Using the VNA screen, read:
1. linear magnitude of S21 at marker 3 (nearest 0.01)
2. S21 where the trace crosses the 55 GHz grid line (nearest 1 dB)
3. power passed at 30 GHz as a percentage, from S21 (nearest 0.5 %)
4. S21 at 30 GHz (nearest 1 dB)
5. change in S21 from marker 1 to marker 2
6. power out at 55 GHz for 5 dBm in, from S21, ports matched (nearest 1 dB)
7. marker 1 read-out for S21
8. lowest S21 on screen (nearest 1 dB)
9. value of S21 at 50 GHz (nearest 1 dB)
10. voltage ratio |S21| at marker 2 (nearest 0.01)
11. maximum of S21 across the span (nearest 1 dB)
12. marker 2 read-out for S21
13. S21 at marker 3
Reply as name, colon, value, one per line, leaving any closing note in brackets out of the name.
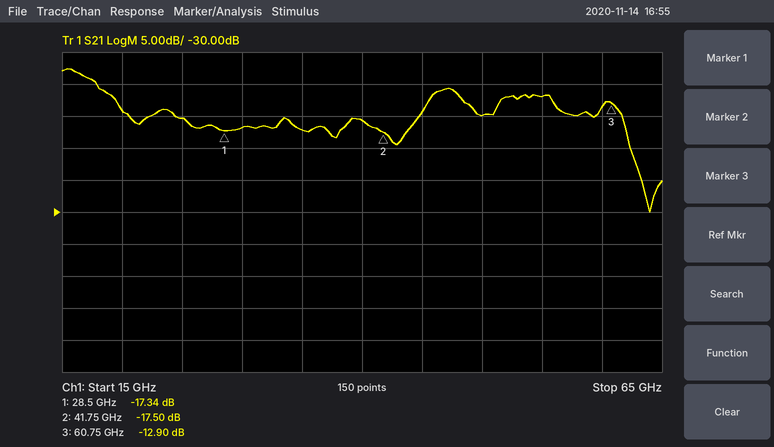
linear magnitude of S21 at marker 3: 0.23
S21 where the trace crosses the 55 GHz grid line: -12 dB
power passed at 30 GHz as a percentage, from S21: 2.0 %
S21 at 30 GHz: -17 dB
change in S21 from marker 1 to marker 2: -0.16 dB
power out at 55 GHz for 5 dBm in, from S21, ports matched: -7 dBm
marker 1 read-out for S21: -17.34 dB
lowest S21 on screen: -30 dB
value of S21 at 50 GHz: -15 dB
voltage ratio |S21| at marker 2: 0.13
maximum of S21 across the span: -8 dB
marker 2 read-out for S21: -17.50 dB
S21 at marker 3: -12.90 dB
